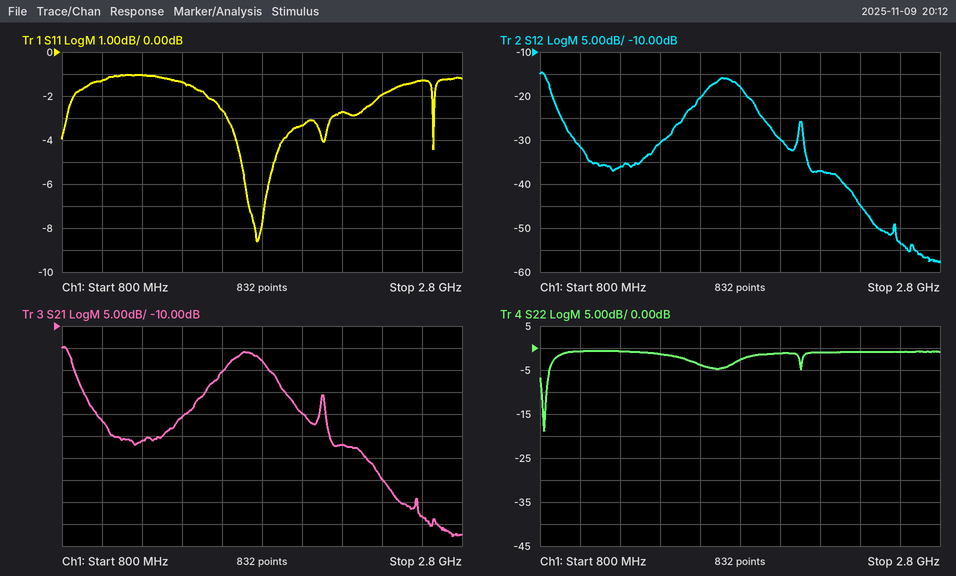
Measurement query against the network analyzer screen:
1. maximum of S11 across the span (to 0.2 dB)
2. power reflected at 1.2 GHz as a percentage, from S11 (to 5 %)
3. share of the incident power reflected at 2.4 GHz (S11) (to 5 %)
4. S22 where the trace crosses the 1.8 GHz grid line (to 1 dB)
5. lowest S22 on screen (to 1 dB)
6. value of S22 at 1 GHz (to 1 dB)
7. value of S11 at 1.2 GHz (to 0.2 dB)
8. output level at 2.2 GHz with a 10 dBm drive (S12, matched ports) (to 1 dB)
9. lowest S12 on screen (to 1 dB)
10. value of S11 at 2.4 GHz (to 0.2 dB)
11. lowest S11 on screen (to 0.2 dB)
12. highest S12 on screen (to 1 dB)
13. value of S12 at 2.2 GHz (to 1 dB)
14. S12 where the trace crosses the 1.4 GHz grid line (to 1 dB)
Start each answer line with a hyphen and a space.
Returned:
- -1.0 dB
- 80 %
- 65 %
- -3 dB
- -19 dB
- -1 dB
- -1.0 dB
- -27 dBm
- -58 dB
- -2.0 dB
- -8.6 dB
- -15 dB
- -37 dB
- -31 dB
